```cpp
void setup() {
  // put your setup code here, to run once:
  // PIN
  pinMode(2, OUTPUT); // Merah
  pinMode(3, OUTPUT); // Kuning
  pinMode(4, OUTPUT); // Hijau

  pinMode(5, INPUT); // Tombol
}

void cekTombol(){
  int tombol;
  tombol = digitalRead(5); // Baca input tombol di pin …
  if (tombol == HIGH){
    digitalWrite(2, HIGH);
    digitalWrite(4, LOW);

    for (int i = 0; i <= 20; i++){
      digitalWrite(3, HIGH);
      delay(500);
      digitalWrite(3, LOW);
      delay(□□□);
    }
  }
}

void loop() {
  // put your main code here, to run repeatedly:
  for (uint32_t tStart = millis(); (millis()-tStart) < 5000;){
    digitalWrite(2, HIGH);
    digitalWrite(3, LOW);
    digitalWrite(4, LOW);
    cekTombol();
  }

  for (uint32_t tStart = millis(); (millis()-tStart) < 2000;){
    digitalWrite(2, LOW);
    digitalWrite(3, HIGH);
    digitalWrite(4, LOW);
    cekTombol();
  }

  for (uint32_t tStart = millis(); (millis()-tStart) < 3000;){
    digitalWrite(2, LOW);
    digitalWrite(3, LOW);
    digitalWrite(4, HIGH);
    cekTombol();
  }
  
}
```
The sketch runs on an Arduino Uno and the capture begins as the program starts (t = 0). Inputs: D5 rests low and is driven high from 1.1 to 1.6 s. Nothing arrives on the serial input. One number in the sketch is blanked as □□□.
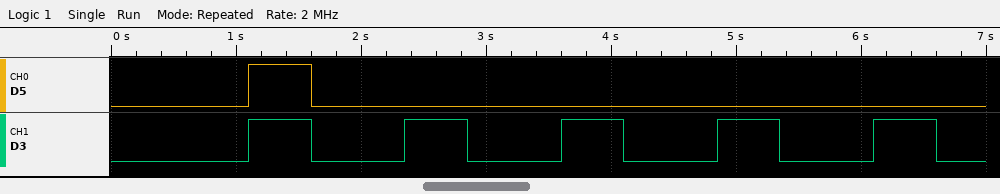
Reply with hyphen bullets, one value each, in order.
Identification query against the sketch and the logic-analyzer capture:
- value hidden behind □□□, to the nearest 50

- 750
